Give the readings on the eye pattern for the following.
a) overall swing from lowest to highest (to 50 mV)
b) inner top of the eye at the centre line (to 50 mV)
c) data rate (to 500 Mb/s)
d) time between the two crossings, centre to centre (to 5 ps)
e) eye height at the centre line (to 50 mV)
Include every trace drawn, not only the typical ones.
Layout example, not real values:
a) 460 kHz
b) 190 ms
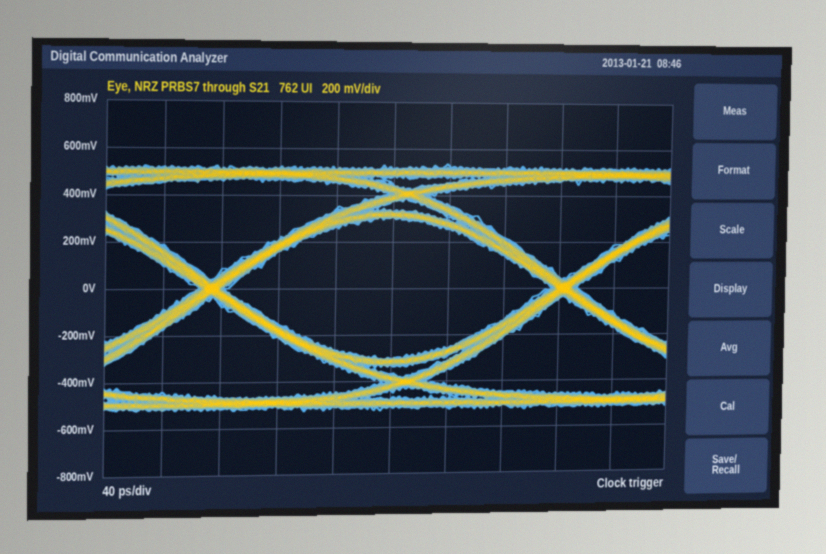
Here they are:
a) 1.05 V
b) 300 mV
c) 4.0 Gb/s
d) 250 ps
e) 600 mV
